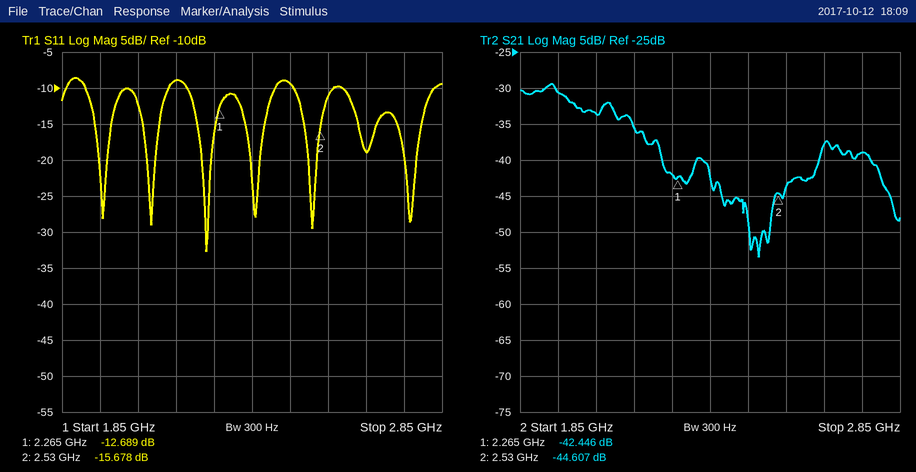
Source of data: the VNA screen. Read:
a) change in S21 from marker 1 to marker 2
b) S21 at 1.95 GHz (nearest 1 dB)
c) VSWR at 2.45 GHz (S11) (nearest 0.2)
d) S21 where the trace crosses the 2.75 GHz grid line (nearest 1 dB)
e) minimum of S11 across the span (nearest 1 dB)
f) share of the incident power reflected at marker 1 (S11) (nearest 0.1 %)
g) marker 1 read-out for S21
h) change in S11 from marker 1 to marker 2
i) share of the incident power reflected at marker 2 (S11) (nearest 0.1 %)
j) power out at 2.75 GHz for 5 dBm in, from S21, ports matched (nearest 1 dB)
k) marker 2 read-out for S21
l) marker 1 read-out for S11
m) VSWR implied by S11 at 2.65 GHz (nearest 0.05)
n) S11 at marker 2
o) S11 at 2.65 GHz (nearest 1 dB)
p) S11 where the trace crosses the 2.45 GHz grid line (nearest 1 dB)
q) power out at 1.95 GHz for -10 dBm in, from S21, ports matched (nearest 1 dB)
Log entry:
-2.161 dB
-31 dB
2.0
-39 dB
-33 dB
5.4 %
-42.446 dB
-2.989 dB
2.7 %
-34 dBm
-44.607 dB
-12.689 dB
1.25
-15.678 dB
-19 dB
-9 dB
-41 dBm
